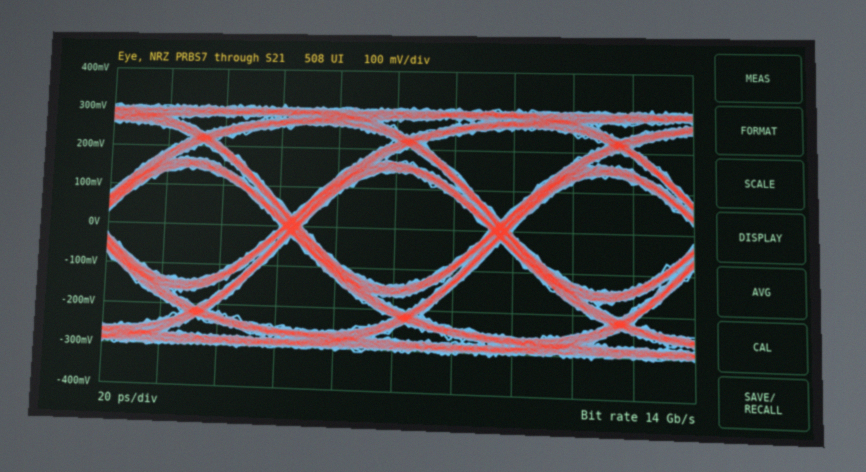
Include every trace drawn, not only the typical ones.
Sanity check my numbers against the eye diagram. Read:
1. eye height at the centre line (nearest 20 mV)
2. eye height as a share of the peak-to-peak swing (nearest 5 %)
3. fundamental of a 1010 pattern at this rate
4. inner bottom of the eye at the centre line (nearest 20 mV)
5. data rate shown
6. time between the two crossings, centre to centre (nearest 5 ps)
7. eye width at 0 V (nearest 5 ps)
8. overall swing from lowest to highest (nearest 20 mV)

280 mV
45 %
7 GHz
-140 mV
14 Gb/s
70 ps
65 ps
620 mV
